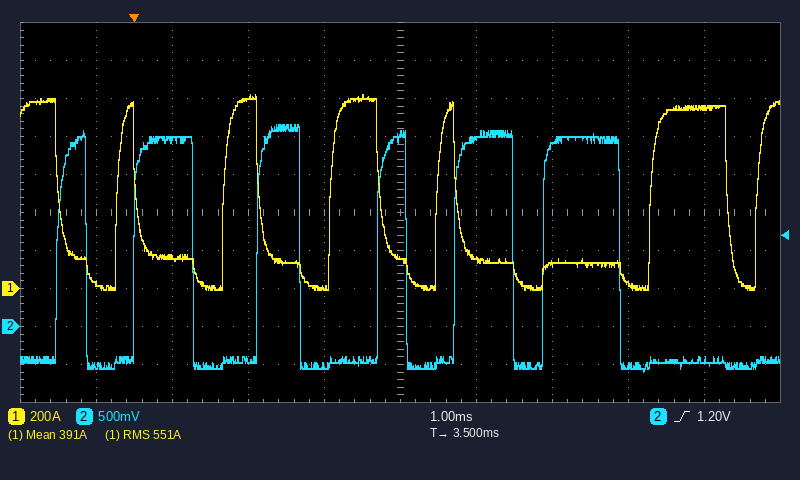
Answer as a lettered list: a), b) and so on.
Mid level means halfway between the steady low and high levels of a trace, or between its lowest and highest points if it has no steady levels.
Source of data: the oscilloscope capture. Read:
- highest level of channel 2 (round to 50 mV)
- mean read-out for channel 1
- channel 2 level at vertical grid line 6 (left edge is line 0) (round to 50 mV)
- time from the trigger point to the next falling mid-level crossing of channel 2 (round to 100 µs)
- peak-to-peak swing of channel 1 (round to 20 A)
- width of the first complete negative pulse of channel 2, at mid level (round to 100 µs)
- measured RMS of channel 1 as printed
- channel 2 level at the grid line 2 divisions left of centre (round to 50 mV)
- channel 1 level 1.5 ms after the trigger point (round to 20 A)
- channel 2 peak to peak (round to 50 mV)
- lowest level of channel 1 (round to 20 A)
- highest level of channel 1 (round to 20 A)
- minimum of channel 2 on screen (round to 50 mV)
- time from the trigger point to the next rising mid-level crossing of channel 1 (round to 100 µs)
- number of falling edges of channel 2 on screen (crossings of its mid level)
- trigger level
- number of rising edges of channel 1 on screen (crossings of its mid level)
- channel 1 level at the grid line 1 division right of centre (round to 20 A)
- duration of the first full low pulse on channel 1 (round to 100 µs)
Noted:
a) 2.65 V
b) 391 A
c) 2.45 V
d) 800 µs
e) 1.02 kA
f) 600 µs
g) 551 A
h) -450 mV
i) 1.00 kA
j) 3.25 V
k) 0 A
l) 1.02 kA
m) -600 mV
n) 1.2 ms
o) 6
p) 1.20 V
q) 6
r) 160 A
s) 800 µs
